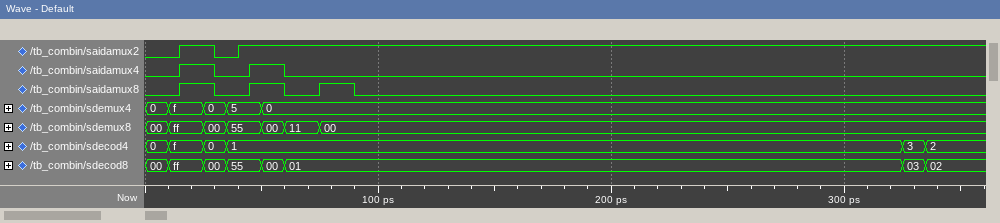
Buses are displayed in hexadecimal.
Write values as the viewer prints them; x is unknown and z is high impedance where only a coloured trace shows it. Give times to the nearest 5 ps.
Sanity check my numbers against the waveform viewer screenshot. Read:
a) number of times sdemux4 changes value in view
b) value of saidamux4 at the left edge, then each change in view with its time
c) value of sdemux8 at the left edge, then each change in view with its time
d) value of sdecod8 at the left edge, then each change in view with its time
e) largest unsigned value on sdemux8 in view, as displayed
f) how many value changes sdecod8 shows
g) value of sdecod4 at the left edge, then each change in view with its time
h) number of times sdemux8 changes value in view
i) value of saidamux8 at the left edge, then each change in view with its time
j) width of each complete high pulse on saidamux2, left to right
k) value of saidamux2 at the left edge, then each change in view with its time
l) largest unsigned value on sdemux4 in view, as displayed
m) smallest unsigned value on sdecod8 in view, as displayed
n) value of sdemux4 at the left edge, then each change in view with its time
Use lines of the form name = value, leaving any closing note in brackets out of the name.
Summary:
number of times sdemux4 changes value in view = 4
value of saidamux4 at the left edge, then each change in view with its time = 0, 1 at 15 ps, 0 at 30 ps, 1 at 45 ps, 0 at 60 ps
value of sdemux8 at the left edge, then each change in view with its time = 00, ff at 10 ps, 00 at 25 ps, 55 at 35 ps, 00 at 50 ps, 11 at 60 ps, 00 at 75 ps
value of sdecod8 at the left edge, then each change in view with its time = 00, ff at 10 ps, 00 at 25 ps, 55 at 35 ps, 00 at 50 ps, 01 at 60 ps, 03 at 325 ps, 02 at 335 ps
largest unsigned value on sdemux8 in view, as displayed = ff
how many value changes sdecod8 shows = 7
value of sdecod4 at the left edge, then each change in view with its time = 0, f at 10 ps, 0 at 25 ps, 1 at 35 ps, 3 at 325 ps, 2 at 335 ps
number of times sdemux8 changes value in view = 6
value of saidamux8 at the left edge, then each change in view with its time = 0, 1 at 15 ps, 0 at 30 ps, 1 at 45 ps, 0 at 60 ps, 1 at 75 ps, 0 at 90 ps
width of each complete high pulse on saidamux2, left to right = 15 ps
value of saidamux2 at the left edge, then each change in view with its time = 0, 1 at 15 ps, 0 at 30 ps, 1 at 40 ps
largest unsigned value on sdemux4 in view, as displayed = f
smallest unsigned value on sdecod8 in view, as displayed = 00
value of sdemux4 at the left edge, then each change in view with its time = 0, f at 10 ps, 0 at 25 ps, 5 at 35 ps, 0 at 50 ps
